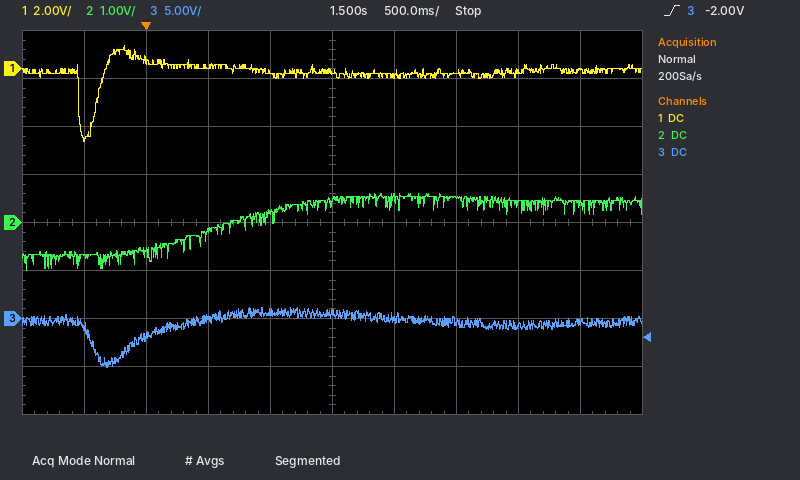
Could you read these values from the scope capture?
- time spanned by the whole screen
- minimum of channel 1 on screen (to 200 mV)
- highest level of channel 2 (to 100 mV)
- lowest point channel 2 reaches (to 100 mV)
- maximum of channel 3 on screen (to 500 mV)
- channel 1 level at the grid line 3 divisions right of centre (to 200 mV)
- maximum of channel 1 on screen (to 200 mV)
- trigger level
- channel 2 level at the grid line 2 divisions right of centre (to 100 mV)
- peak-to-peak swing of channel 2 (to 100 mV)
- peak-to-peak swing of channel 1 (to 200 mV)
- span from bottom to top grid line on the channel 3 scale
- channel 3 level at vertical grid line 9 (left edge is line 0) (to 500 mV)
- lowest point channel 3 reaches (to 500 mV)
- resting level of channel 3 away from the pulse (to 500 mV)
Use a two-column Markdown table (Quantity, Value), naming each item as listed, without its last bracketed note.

| Quantity | Value |
|---|---|
| time spanned by the whole screen | 5 s |
| minimum of channel 1 on screen | -3.0 V |
| highest level of channel 2 | 600 mV |
| lowest point channel 2 reaches | -1.0 V |
| maximum of channel 3 on screen | 1.0 V |
| channel 1 level at the grid line 3 divisions right of centre | -200 mV |
| maximum of channel 1 on screen | 1.0 V |
| trigger level | -2.00 V |
| channel 2 level at the grid line 2 divisions right of centre | 500 mV |
| peak-to-peak swing of channel 2 | 1.6 V |
| peak-to-peak swing of channel 1 | 4.0 V |
| span from bottom to top grid line on the channel 3 scale | 40 V |
| channel 3 level at vertical grid line 9 (left edge is line 0) | -500 mV |
| lowest point channel 3 reaches | -5.0 V |
| resting level of channel 3 away from the pulse | -500 mV |
